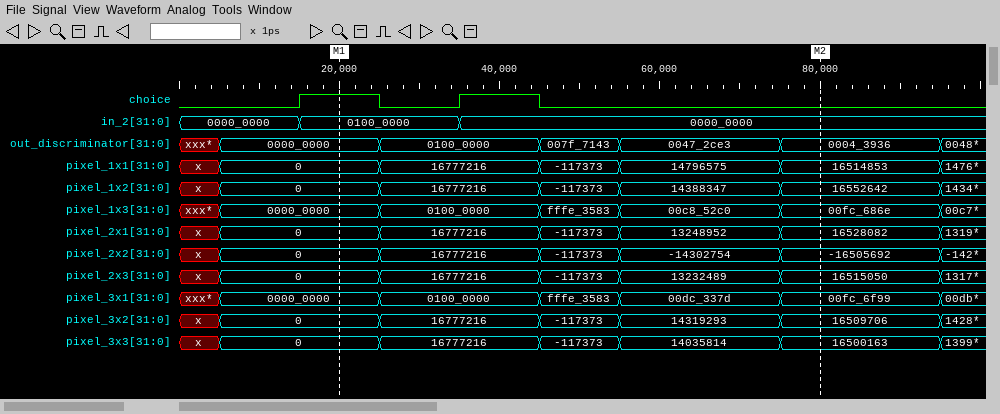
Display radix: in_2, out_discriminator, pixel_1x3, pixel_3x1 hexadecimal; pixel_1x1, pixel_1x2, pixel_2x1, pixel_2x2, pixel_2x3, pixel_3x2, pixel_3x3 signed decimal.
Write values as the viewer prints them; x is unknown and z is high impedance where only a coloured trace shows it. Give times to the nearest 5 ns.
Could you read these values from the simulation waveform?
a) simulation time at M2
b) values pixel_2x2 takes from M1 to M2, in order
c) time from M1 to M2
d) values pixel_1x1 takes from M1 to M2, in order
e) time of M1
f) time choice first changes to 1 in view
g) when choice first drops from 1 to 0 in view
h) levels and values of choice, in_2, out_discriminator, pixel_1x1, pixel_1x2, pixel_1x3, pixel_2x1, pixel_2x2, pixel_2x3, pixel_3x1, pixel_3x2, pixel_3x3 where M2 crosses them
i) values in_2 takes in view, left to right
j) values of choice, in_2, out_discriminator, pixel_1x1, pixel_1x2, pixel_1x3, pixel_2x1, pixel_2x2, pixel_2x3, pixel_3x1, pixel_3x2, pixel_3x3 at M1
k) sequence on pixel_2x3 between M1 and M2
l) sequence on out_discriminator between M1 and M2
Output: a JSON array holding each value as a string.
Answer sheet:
["80 ns", "0, 16777216, -117373, -14302754, -16505692", "60 ns", "0, 16777216, -117373, 14796575, 16514853", "20 ns", "15 ns", "25 ns", "choice=0, in_2=0000_0000, out_discriminator=0004_3936, pixel_1x1=16514853, pixel_1x2=16552642, pixel_1x3=00fc_686e, pixel_2x1=16528082, pixel_2x2=-16505692, pixel_2x3=16515050, pixel_3x1=00fc_6f99, pixel_3x2=16509706, pixel_3x3=16500163", "0000_0000, 0100_0000, 0000_0000", "choice=1, in_2=0100_0000, out_discriminator=0000_0000, pixel_1x1=0, pixel_1x2=0, pixel_1x3=0000_0000, pixel_2x1=0, pixel_2x2=0, pixel_2x3=0, pixel_3x1=0000_0000, pixel_3x2=0, pixel_3x3=0", "0, 16777216, -117373, 13232489, 16515050", "0000_0000, 0100_0000, 007f_7143, 0047_2ce3, 0004_3936"]
